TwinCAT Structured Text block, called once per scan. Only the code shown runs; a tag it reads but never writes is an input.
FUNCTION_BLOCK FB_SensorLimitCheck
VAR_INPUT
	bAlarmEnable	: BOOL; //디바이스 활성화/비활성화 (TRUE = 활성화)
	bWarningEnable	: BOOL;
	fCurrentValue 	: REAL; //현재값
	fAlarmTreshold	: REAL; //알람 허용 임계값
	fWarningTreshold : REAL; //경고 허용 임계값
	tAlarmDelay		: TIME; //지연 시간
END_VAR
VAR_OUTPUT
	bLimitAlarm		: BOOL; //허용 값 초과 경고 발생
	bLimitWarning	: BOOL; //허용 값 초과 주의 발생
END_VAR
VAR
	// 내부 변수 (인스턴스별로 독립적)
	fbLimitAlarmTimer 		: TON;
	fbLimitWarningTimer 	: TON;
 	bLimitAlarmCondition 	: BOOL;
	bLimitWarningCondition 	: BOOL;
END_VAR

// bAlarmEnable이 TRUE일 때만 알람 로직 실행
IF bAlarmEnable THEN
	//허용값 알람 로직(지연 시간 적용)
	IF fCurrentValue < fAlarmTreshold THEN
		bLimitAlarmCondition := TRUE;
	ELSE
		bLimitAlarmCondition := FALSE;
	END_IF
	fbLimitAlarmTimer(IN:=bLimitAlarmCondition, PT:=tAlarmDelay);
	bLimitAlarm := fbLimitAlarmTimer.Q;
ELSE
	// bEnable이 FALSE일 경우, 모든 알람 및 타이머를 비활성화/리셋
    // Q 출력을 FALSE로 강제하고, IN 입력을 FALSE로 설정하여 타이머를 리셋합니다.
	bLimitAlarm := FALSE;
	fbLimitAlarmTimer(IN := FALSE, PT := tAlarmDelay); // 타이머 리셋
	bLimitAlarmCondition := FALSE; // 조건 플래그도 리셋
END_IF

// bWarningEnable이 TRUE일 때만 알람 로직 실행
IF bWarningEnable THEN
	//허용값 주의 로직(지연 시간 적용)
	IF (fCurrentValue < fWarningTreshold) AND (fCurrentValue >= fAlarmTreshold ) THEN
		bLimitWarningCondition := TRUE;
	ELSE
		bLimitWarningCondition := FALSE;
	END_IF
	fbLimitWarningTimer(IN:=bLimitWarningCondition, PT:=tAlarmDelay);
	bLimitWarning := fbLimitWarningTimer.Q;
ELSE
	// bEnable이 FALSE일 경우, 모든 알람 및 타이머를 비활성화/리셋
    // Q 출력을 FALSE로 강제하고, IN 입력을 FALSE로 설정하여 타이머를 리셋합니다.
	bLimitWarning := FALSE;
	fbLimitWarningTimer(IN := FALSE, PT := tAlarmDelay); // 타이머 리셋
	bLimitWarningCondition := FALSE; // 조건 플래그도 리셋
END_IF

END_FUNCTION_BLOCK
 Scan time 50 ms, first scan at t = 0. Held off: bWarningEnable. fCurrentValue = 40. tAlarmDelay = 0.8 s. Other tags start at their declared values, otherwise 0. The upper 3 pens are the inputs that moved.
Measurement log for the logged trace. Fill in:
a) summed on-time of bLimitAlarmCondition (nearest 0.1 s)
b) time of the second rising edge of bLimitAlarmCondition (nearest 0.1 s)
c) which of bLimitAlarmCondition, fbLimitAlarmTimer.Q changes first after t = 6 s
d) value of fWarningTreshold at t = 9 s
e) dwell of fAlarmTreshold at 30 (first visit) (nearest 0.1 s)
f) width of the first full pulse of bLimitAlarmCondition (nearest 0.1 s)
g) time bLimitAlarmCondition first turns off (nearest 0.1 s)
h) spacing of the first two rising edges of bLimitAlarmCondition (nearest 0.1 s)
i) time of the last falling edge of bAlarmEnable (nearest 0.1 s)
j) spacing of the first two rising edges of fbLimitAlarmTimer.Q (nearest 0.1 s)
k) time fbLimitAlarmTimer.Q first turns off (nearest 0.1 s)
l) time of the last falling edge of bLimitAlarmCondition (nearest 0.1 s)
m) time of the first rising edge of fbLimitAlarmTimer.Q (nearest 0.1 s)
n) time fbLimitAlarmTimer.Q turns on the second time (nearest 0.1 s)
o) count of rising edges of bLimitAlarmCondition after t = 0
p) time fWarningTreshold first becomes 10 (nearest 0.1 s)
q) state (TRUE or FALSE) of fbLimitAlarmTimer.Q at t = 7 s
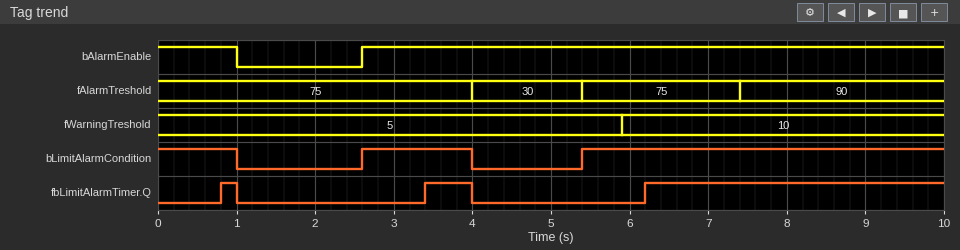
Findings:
7.0 s
5.4 s
fbLimitAlarmTimer.Q
10
1.4 s
1.4 s
1.0 s
2.8 s
1.0 s
2.6 s
1.0 s
4.0 s
0.8 s
3.4 s
2
5.9 s
TRUE
